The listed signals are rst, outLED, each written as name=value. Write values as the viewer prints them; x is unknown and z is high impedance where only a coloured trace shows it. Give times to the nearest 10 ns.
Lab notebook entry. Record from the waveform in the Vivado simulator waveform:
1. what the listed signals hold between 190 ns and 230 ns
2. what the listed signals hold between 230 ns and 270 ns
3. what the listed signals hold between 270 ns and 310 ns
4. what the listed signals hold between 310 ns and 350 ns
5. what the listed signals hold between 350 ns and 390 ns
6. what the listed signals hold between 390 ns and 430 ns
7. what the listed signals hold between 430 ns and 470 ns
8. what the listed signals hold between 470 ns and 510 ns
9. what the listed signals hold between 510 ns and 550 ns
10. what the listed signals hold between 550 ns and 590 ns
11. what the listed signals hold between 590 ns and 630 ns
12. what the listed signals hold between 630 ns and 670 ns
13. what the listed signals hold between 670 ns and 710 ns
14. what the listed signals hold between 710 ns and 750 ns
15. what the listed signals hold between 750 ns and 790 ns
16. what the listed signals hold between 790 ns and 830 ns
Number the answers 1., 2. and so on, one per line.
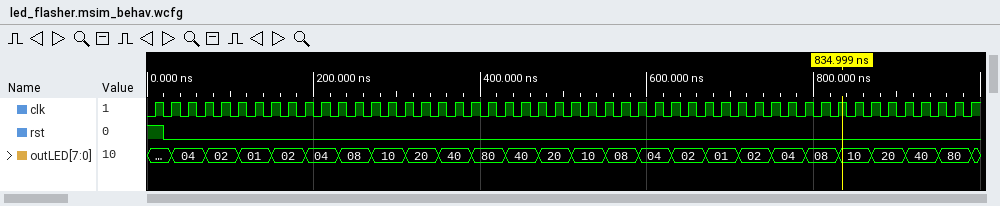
1. rst=0, outLED=04
2. rst=0, outLED=08
3. rst=0, outLED=10
4. rst=0, outLED=20
5. rst=0, outLED=40
6. rst=0, outLED=80
7. rst=0, outLED=40
8. rst=0, outLED=20
9. rst=0, outLED=10
10. rst=0, outLED=08
11. rst=0, outLED=04
12. rst=0, outLED=02
13. rst=0, outLED=01
14. rst=0, outLED=02
15. rst=0, outLED=04
16. rst=0, outLED=08
